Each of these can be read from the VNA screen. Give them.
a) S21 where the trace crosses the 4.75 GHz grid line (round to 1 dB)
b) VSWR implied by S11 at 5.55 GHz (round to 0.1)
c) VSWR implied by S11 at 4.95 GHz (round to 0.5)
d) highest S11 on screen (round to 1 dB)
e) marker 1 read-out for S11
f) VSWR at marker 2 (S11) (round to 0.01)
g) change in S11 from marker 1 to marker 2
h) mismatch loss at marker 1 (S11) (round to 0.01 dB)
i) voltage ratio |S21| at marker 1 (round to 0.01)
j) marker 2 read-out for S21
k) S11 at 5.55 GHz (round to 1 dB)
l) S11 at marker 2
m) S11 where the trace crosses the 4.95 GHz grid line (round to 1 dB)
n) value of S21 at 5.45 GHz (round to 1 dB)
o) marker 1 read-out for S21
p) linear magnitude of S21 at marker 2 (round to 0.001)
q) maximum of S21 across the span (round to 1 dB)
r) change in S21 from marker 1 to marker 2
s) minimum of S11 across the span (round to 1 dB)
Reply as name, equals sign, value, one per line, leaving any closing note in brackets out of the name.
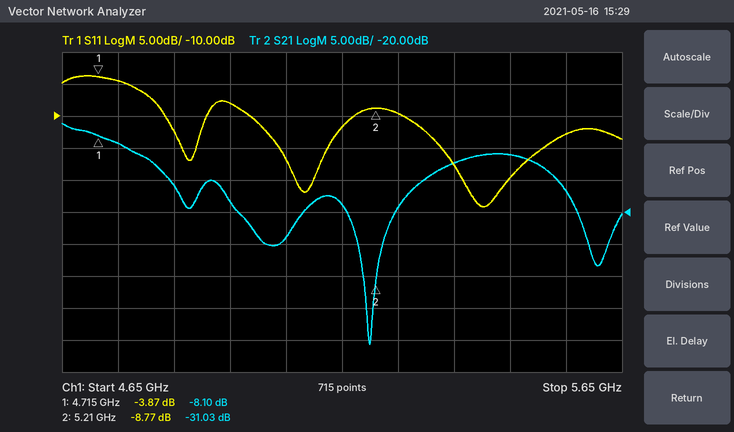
S21 where the trace crosses the 4.75 GHz grid line = -9 dB
VSWR implied by S11 at 5.55 GHz = 1.6
VSWR implied by S11 at 4.95 GHz = 2.5
highest S11 on screen = -4 dB
marker 1 read-out for S11 = -3.87 dB
VSWR at marker 2 (S11) = 2.15
change in S11 from marker 1 to marker 2 = -4.90 dB
mismatch loss at marker 1 (S11) = 2.29 dB
voltage ratio |S21| at marker 1 = 0.39
marker 2 read-out for S21 = -31.03 dB
S11 at 5.55 GHz = -13 dB
S11 at marker 2 = -8.77 dB
S11 where the trace crosses the 4.95 GHz grid line = -8 dB
value of S21 at 5.45 GHz = -11 dB
marker 1 read-out for S21 = -8.10 dB
linear magnitude of S21 at marker 2 = 0.028
maximum of S21 across the span = -6 dB
change in S21 from marker 1 to marker 2 = -22.93 dB
minimum of S11 across the span = -24 dB
